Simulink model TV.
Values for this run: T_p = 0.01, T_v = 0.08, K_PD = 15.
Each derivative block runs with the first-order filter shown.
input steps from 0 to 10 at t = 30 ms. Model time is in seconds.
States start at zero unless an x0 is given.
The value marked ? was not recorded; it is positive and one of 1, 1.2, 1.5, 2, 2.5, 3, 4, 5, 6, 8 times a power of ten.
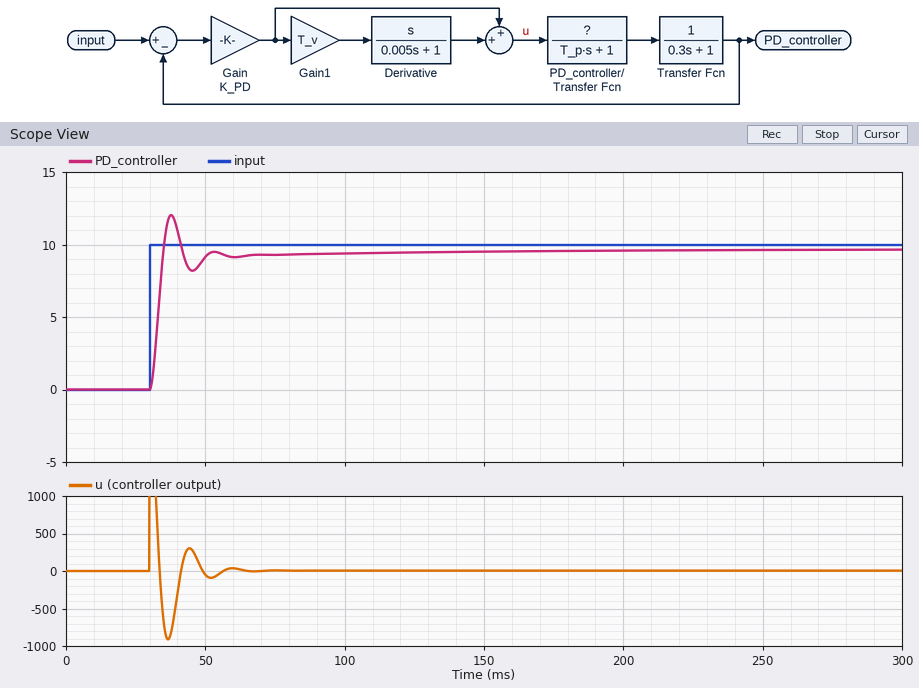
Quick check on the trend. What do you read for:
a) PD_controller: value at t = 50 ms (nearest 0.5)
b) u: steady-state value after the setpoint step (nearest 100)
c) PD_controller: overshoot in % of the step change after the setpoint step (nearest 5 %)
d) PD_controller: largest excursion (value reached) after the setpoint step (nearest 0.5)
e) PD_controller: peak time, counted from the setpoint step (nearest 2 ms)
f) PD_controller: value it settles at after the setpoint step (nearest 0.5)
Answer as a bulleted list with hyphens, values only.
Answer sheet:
- 9.0
- 0
- 25 %
- 12.0
- 8 ms
- 9.5
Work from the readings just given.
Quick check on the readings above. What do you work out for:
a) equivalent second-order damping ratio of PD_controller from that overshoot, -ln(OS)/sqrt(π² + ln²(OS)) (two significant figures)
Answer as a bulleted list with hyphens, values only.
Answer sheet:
- 0.40
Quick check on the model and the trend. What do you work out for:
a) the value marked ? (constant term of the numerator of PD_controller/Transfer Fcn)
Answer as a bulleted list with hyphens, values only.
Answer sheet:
- 2
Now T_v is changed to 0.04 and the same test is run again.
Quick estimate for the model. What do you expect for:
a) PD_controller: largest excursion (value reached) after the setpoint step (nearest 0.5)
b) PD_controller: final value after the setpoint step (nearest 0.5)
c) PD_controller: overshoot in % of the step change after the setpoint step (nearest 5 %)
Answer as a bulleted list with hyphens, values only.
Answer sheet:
- 10.5
- 9.5
- 10 %
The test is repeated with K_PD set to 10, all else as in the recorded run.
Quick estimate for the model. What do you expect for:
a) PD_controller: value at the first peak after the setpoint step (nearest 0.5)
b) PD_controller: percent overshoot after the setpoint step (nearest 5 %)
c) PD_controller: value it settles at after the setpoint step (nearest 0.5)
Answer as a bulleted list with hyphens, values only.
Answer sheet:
- 11.0
- 15 %
- 9.5
